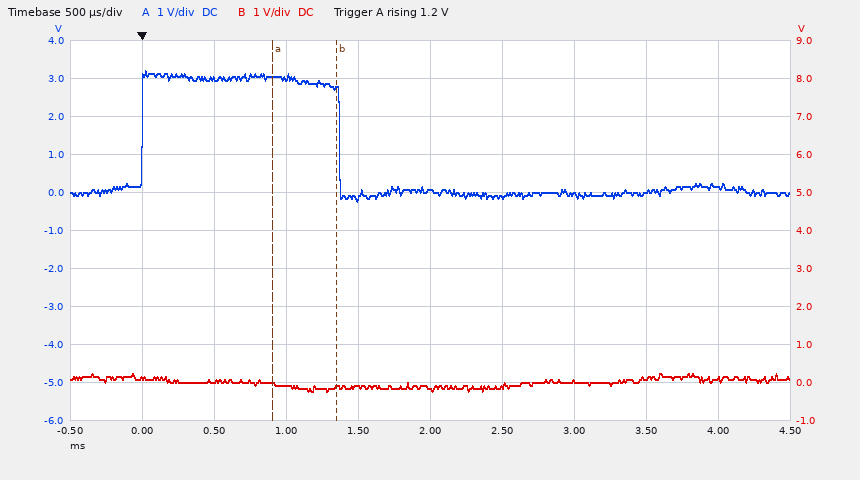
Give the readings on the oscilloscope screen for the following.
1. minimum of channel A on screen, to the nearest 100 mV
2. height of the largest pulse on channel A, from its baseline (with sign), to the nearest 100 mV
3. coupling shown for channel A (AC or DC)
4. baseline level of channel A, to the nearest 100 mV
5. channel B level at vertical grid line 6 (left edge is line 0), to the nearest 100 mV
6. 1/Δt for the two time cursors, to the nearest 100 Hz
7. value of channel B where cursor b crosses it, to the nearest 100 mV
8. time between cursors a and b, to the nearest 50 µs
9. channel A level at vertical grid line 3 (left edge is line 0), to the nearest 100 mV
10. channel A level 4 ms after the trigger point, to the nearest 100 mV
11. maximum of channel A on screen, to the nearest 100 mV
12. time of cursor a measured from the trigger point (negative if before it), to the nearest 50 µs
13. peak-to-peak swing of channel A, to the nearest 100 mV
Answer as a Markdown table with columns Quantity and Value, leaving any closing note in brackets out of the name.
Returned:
| Quantity | Value |
|---|---|
| minimum of channel A on screen, to the nearest 100 mV | -200 mV |
| height of the largest pulse on channel A, from its baseline (with sign), to the nearest 100 mV | +3.2 V |
| coupling shown for channel A | DC |
| baseline level of channel A, to the nearest 100 mV | 0.0 V |
| channel B level at vertical grid line 6 (left edge is line 0), to the nearest 100 mV | -100 mV |
| 1/Δt for the two time cursors, to the nearest 100 Hz | 2.2 kHz |
| value of channel B where cursor b crosses it, to the nearest 100 mV | -100 mV |
| time between cursors a and b, to the nearest 50 µs | 450 µs |
| channel A level at vertical grid line 3 (left edge is line 0), to the nearest 100 mV | 3.0 V |
| channel A level 4 ms after the trigger point, to the nearest 100 mV | 100 mV |
| maximum of channel A on screen, to the nearest 100 mV | 3.2 V |
| time of cursor a measured from the trigger point (negative if before it), to the nearest 50 µs | +900 µs |
| peak-to-peak swing of channel A, to the nearest 100 mV | 3.4 V |
